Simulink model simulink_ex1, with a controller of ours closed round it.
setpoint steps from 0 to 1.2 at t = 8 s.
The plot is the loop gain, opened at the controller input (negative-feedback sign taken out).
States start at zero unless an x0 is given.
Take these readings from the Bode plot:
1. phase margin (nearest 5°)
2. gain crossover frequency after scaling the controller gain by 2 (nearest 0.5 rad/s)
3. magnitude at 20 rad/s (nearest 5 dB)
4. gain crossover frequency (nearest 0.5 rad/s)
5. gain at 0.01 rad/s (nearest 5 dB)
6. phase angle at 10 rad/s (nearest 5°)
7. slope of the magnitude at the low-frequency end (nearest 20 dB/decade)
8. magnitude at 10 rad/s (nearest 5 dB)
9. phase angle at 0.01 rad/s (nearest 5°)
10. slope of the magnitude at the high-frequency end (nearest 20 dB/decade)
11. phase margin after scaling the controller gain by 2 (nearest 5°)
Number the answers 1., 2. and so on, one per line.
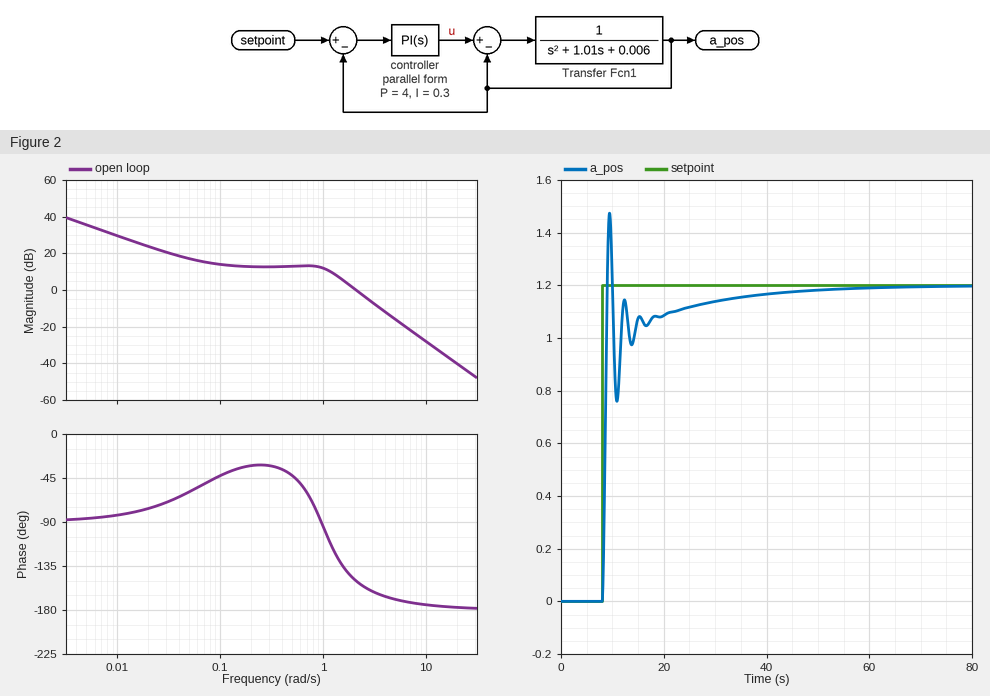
1. 30°
2. 3.0 rad/s
3. -40 dB
4. 2.0 rad/s
5. 30 dB
6. -175°
7. -20 dB/decade
8. -30 dB
9. -85°
10. -40 dB/decade
11. 20°
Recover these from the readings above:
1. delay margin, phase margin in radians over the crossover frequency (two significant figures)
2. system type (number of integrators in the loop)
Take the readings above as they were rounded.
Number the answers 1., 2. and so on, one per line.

1. 0.26 s
2. 1
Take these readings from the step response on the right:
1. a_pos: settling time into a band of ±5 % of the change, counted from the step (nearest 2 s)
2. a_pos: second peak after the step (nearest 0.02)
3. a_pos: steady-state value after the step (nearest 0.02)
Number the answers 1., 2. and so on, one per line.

1. 22 s
2. 1.14
3. 1.20
